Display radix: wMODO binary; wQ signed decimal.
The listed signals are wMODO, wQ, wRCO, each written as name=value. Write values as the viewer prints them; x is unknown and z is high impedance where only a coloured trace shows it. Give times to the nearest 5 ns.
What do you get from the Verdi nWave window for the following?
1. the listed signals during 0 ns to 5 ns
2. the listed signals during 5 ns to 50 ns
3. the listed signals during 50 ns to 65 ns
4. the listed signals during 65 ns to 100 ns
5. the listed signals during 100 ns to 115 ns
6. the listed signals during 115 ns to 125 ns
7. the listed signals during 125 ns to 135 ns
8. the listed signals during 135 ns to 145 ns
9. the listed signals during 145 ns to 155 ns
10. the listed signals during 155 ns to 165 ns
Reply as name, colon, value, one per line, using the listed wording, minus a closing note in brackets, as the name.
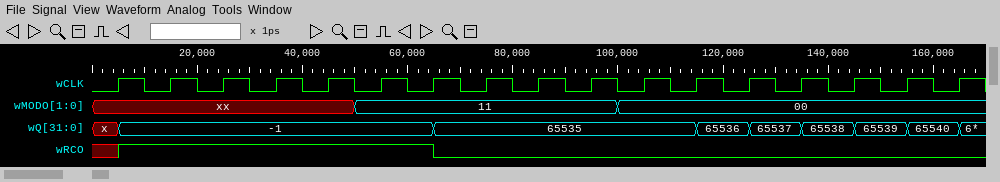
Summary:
the listed signals during 0 ns to 5 ns: wMODO=xx, wQ=x, wRCO=x
the listed signals during 5 ns to 50 ns: wMODO=xx, wQ=-1, wRCO=1
the listed signals during 50 ns to 65 ns: wMODO=11, wQ=-1, wRCO=1
the listed signals during 65 ns to 100 ns: wMODO=11, wQ=65535, wRCO=0
the listed signals during 100 ns to 115 ns: wMODO=00, wQ=65535, wRCO=0
the listed signals during 115 ns to 125 ns: wMODO=00, wQ=65536, wRCO=0
the listed signals during 125 ns to 135 ns: wMODO=00, wQ=65537, wRCO=0
the listed signals during 135 ns to 145 ns: wMODO=00, wQ=65538, wRCO=0
the listed signals during 145 ns to 155 ns: wMODO=00, wQ=65539, wRCO=0
the listed signals during 155 ns to 165 ns: wMODO=00, wQ=65540, wRCO=0
